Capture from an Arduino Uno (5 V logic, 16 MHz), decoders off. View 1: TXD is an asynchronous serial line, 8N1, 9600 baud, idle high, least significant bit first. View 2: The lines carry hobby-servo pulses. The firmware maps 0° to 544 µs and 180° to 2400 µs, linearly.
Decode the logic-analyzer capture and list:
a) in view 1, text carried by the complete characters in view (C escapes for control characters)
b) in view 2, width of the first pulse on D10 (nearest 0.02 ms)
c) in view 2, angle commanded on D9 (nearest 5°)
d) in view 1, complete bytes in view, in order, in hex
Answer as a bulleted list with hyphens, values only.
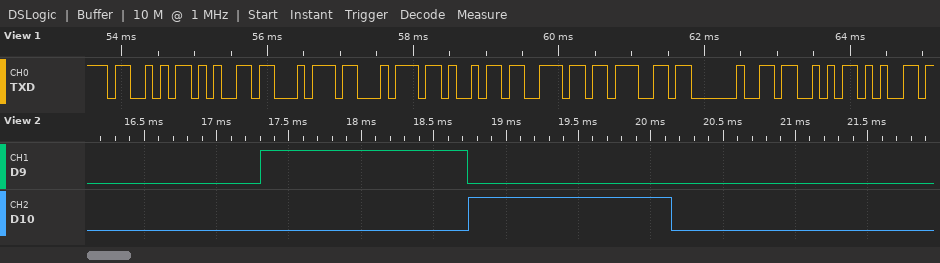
- "Setting Se"
- 1.40 ms
- 85°
- 53 65 74 74 69 6E 67 20 53 65
